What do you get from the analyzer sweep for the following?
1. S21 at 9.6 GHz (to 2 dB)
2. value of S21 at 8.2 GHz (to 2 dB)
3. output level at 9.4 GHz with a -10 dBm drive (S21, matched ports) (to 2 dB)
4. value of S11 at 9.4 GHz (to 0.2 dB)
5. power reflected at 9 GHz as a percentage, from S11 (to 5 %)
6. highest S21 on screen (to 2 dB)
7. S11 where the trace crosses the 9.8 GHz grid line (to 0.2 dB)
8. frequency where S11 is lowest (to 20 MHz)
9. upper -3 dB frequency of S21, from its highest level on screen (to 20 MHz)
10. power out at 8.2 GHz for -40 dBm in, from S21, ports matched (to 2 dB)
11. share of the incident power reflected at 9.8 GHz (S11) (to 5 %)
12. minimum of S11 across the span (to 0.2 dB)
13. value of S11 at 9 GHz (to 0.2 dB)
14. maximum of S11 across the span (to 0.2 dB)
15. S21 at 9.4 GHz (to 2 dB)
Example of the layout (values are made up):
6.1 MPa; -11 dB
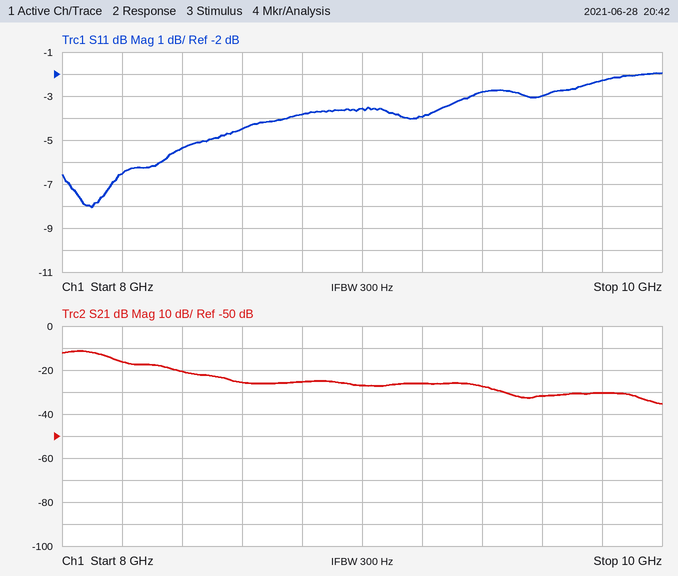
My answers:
-32 dB; -16 dB; -38 dBm; -2.8 dB; 45 %; -12 dB; -2.2 dB; 8.10 GHz; 8.16 GHz; -56 dBm; 60 %; -8.0 dB; -3.6 dB; -2.0 dB; -28 dB
